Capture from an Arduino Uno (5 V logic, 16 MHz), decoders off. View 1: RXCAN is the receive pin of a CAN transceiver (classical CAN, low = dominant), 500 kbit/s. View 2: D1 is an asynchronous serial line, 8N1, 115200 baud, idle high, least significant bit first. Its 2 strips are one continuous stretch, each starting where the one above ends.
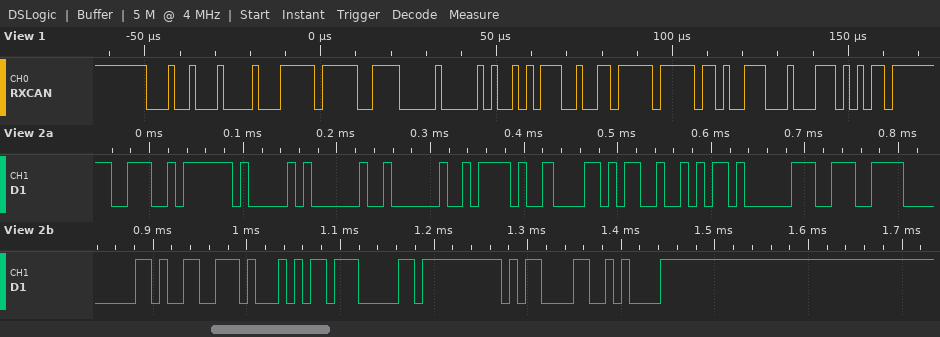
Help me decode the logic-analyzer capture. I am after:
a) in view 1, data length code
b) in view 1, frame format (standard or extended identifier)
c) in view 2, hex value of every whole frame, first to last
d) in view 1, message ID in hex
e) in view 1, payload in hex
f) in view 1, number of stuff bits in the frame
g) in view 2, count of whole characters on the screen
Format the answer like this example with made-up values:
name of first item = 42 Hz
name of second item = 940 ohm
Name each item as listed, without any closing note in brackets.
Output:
in view 1, data length code = 8
in view 1, frame format = standard
in view 2, hex value of every whole frame, first to last = 0x4E 0x41 0x20 0x20 0x2F 0x58 0x52 0x81 0xCE 0x00 0x99 0x51 0x07 0xFF 0x0D 0x0A
in view 1, message ID in hex = 0x122
in view 1, payload in hex = FF DE 00 25 72 6F FF 4E
in view 1, number of stuff bits in the frame = 6
in view 2, count of whole characters on the screen = 16
